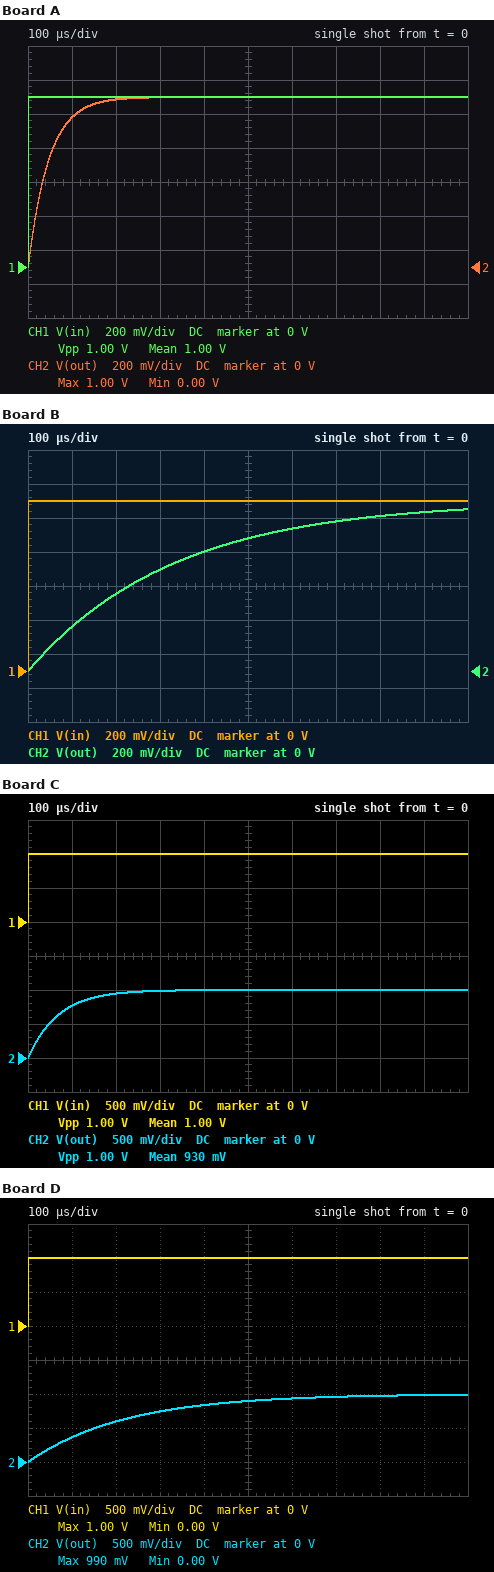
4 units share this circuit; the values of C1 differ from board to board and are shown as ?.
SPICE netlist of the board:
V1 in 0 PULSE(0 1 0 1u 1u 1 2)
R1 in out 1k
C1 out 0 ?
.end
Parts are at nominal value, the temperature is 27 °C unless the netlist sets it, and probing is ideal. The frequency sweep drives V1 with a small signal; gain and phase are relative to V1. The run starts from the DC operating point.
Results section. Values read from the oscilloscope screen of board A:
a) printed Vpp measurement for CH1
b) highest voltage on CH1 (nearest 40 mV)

1.00 V
1.00 V
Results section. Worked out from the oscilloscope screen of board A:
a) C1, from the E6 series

47 nF
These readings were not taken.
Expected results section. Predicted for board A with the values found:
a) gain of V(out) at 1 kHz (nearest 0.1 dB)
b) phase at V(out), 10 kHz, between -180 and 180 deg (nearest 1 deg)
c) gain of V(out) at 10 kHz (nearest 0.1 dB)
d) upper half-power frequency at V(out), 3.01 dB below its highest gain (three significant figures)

-0.4 dB
-71 deg
-9.9 dB
3.39 kHz
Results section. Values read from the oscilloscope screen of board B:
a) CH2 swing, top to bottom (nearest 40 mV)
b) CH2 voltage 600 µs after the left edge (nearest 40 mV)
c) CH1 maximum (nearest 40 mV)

960 mV
840 mV
1.00 V
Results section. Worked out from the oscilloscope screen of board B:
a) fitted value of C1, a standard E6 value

330 nF
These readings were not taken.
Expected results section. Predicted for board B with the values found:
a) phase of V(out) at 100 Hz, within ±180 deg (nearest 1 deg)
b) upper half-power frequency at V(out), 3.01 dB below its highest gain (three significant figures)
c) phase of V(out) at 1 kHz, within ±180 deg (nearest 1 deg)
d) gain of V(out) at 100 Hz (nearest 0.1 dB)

-12 deg
482 Hz
-64 deg
-0.2 dB
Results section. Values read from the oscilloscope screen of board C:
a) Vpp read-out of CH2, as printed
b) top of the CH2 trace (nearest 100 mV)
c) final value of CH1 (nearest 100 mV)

1.00 V
1.0 V
1.0 V
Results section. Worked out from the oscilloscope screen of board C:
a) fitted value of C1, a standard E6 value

68 nF
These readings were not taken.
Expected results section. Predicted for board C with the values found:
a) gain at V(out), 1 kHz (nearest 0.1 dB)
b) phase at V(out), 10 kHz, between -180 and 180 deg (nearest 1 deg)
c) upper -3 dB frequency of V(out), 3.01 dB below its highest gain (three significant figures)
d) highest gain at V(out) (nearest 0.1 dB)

-0.7 dB
-77 deg
2.34 kHz
0 dB
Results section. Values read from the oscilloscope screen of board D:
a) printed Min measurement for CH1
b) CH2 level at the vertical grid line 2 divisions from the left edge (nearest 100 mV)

0.00 V
600 mV
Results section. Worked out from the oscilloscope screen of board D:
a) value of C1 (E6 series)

220 nF
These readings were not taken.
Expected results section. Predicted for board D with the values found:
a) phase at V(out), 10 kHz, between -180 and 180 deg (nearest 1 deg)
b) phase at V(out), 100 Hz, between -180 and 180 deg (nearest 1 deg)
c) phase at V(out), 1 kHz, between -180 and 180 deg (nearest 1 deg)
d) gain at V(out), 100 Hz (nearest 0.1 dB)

-86 deg
-8 deg
-54 deg
-0.1 dB
